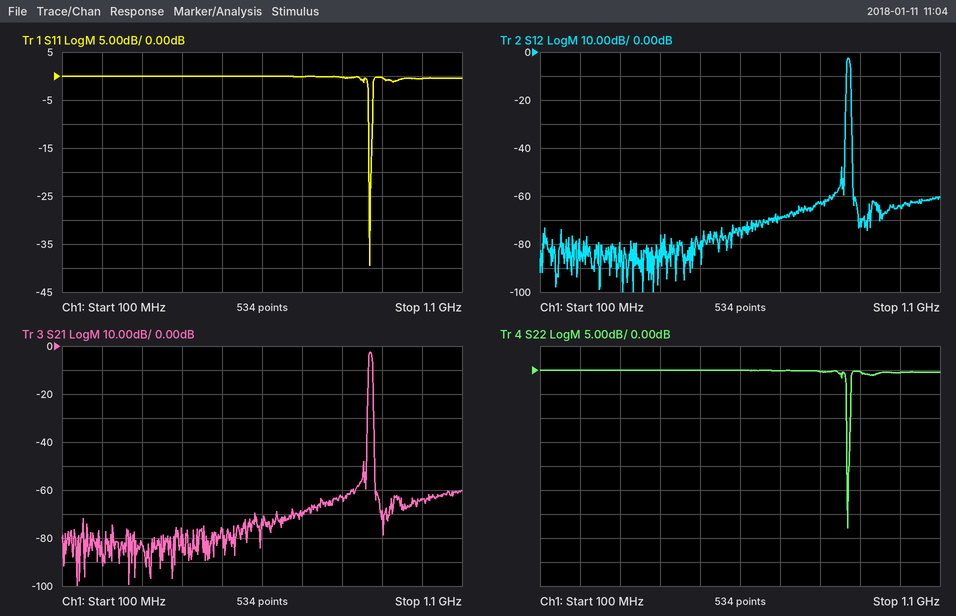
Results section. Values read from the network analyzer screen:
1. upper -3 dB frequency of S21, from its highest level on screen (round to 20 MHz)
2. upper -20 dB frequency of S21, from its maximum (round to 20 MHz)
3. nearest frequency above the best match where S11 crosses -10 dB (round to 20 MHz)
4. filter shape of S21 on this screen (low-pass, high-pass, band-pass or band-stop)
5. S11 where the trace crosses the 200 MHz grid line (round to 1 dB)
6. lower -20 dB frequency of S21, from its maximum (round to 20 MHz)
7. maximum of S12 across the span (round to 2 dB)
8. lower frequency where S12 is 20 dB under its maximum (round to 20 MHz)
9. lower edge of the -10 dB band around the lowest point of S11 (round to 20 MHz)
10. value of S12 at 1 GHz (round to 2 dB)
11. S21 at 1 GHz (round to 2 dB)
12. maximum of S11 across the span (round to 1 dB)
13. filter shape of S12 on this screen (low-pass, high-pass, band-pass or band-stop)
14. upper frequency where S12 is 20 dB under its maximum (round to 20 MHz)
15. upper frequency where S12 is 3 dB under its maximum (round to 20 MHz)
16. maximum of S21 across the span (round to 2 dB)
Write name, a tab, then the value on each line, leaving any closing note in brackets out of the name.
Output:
upper -3 dB frequency of S21, from its highest level on screen	880 MHz
upper -20 dB frequency of S21, from its maximum	880 MHz
nearest frequency above the best match where S11 crosses -10 dB	880 MHz
filter shape of S21 on this screen	band-pass
S11 where the trace crosses the 200 MHz grid line	0 dB
lower -20 dB frequency of S21, from its maximum	860 MHz
maximum of S12 across the span	-2 dB
lower frequency where S12 is 20 dB under its maximum	860 MHz
lower edge of the -10 dB band around the lowest point of S11	860 MHz
value of S12 at 1 GHz	-64 dB
S21 at 1 GHz	-64 dB
maximum of S11 across the span	0 dB
filter shape of S12 on this screen	band-pass
upper frequency where S12 is 20 dB under its maximum	880 MHz
upper frequency where S12 is 3 dB under its maximum	880 MHz
maximum of S21 across the span	-2 dB
